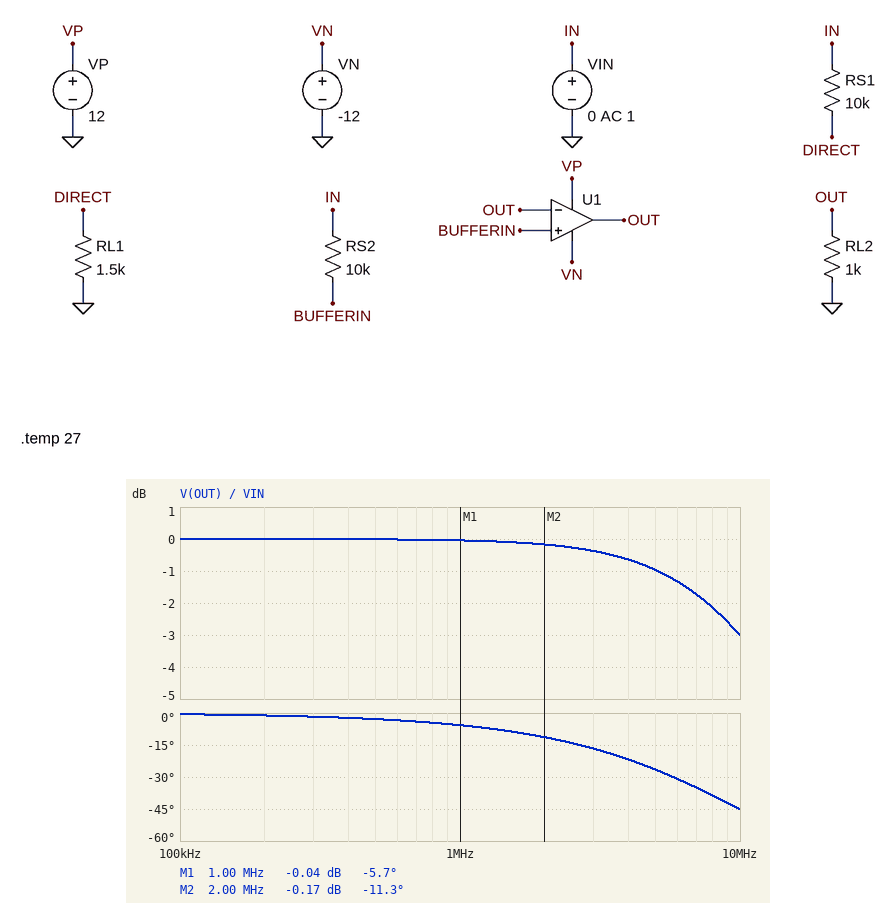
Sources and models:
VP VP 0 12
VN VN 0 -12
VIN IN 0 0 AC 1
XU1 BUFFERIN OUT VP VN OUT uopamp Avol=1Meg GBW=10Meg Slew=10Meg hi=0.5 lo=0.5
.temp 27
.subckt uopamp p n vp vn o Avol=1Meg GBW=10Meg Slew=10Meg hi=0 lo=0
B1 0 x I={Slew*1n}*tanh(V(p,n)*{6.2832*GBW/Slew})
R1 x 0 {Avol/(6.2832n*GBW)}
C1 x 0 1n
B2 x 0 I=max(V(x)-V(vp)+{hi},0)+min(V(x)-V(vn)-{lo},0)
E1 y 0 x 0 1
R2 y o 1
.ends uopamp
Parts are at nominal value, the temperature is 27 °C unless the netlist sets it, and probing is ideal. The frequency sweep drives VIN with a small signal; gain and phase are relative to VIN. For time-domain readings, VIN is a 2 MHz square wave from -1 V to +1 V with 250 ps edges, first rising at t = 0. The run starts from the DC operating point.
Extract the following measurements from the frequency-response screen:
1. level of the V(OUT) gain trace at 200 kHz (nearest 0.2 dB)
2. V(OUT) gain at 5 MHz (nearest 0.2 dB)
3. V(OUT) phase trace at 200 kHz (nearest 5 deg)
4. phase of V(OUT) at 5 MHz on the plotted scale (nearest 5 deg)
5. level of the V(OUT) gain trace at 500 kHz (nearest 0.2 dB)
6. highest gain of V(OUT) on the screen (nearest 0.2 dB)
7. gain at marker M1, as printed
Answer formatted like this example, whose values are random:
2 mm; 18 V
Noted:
0 dB; -1.0 dB; 0 deg; -25 deg; 0 dB; 0 dB; -0.04 dB
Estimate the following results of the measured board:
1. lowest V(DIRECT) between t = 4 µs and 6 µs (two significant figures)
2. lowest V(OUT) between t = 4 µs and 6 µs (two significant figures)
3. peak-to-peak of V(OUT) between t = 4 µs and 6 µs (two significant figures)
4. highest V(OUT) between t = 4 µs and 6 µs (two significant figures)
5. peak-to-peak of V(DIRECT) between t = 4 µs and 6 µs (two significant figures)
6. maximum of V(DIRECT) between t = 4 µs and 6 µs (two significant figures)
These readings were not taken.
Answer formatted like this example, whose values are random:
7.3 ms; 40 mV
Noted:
-130 mV; -1.0 V; 2.0 V; 1.0 V; 260 mV; 130 mV
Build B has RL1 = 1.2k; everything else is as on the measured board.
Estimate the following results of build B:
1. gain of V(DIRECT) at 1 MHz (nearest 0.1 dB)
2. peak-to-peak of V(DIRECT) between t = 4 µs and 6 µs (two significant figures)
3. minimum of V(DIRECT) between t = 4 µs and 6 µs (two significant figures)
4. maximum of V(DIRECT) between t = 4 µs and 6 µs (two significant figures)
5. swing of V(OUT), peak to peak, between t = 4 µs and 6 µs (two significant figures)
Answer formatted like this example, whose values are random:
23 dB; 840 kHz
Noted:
-19.4 dB; 210 mV; -110 mV; 110 mV; 2.0 V
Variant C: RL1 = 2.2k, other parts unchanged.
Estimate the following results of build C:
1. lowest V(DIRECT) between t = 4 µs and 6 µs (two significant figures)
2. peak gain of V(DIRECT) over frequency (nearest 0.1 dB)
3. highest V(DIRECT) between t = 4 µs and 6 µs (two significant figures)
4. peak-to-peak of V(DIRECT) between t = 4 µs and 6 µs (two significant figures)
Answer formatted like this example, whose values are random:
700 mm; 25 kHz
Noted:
-180 mV; -14.9 dB; 180 mV; 360 mV
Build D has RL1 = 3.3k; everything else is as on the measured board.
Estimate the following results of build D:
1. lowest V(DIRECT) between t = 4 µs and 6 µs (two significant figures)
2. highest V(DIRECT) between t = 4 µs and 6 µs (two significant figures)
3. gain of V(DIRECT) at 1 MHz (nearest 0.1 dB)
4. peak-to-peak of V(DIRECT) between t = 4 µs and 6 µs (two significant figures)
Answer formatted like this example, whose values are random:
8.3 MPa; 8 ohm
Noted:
-250 mV; 250 mV; -12.1 dB; 500 mV
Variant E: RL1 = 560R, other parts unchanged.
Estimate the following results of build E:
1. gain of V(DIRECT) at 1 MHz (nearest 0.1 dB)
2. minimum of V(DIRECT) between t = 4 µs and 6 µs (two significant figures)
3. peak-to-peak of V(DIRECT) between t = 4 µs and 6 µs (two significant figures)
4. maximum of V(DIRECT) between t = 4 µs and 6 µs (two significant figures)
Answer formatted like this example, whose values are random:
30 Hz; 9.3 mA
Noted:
-25.5 dB; -53 mV; 110 mV; 53 mV
